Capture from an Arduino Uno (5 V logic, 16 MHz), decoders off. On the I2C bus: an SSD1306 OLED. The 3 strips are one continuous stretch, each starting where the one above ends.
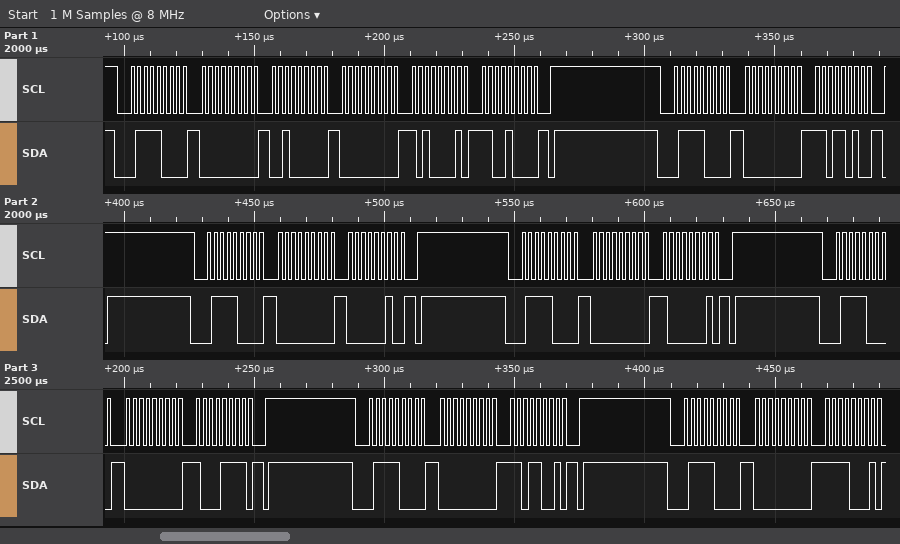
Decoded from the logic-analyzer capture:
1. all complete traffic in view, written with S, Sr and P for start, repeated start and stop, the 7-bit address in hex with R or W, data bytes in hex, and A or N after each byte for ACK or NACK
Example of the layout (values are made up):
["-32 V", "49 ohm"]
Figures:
["S 3CW A 00 A 20 A 00 A A1 A C8 A P S 3CW A 00 A DA A P S 3CW A 00 A 02 A P S 3CW A 00 A 81 A P S 3CW A 00 A 8F A P S 3CW A 00 A D9 A P S 3CW A 00 A F1 A"]
